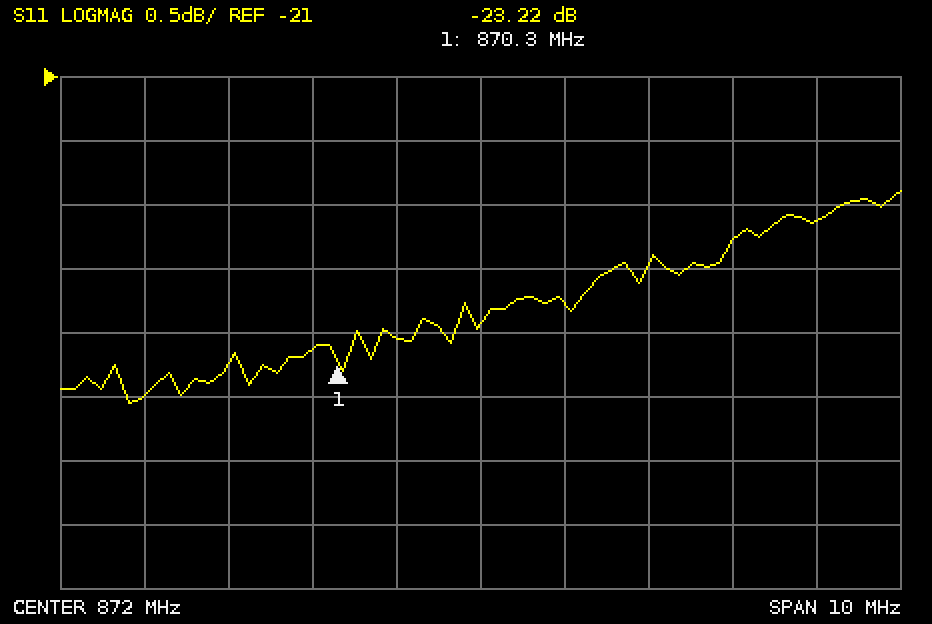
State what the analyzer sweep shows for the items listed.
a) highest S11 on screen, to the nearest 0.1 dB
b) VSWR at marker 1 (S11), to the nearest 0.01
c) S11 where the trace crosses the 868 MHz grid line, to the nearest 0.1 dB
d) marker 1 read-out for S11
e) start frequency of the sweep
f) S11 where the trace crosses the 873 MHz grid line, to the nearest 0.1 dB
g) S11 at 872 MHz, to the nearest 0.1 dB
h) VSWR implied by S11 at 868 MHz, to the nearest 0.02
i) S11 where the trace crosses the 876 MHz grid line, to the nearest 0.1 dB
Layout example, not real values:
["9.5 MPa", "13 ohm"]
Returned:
["-21.9 dB", "1.15", "-23.5 dB", "-23.22 dB", "867 MHz", "-22.8 dB", "-22.9 dB", "1.14", "-22.1 dB"]
